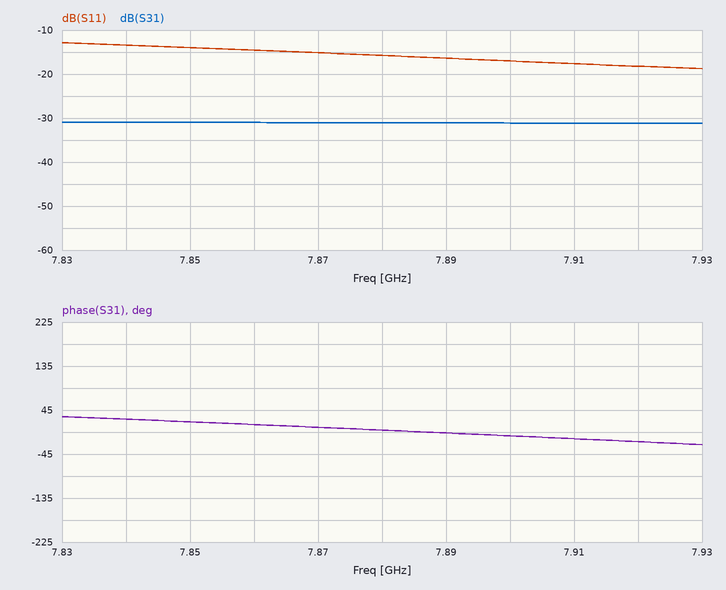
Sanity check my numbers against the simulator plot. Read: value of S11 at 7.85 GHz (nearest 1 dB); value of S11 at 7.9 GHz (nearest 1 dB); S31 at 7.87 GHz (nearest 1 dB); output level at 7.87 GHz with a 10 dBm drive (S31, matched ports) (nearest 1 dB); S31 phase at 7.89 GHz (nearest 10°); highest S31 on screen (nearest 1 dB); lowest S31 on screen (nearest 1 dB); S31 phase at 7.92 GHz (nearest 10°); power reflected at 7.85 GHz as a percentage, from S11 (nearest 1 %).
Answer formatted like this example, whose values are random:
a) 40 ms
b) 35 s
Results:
a) -14 dB
b) -17 dB
c) -31 dB
d) -21 dBm
e) 0°
f) -31 dB
g) -31 dB
h) -20°
i) 4 %
